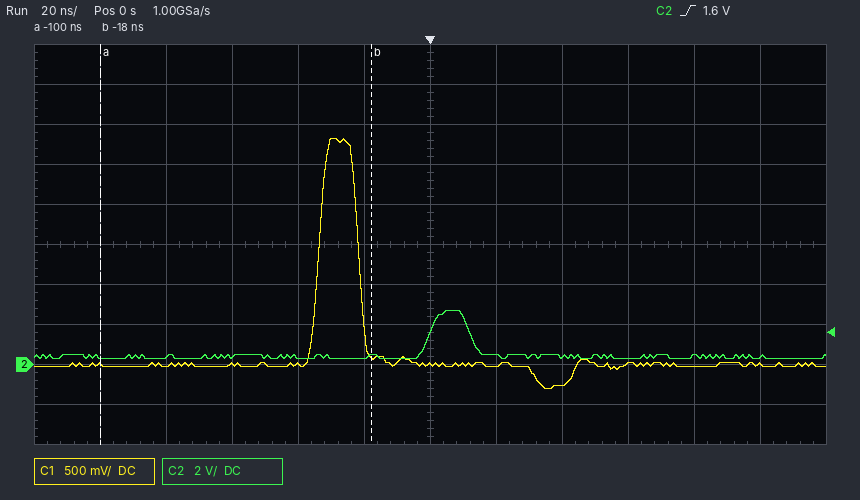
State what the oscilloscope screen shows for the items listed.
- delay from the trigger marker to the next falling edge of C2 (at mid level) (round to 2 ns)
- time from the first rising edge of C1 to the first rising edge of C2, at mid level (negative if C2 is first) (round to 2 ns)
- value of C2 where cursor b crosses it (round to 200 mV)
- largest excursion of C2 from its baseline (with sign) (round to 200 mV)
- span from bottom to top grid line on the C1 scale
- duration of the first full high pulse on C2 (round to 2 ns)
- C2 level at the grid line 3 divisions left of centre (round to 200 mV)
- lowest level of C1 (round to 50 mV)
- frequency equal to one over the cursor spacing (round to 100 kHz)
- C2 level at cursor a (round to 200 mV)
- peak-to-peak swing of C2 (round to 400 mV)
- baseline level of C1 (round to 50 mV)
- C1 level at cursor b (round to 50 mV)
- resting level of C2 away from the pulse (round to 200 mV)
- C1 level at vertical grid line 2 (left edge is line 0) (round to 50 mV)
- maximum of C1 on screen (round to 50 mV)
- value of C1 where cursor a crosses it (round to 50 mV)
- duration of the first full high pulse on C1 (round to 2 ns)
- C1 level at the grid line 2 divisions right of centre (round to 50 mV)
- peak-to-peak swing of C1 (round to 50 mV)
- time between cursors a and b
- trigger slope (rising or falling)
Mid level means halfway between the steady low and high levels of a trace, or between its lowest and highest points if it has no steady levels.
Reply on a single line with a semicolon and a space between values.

12 ns; +34 ns; 400 mV; +2.4 V; 5 V; 12 ns; 400 mV; -300 mV; 12.2 MHz; 400 mV; 2.4 V; 0 mV; 100 mV; 400 mV; 0 mV; 2.80 V; 0 mV; 12 ns; -250 mV; 3.10 V; 82 ns; rising
